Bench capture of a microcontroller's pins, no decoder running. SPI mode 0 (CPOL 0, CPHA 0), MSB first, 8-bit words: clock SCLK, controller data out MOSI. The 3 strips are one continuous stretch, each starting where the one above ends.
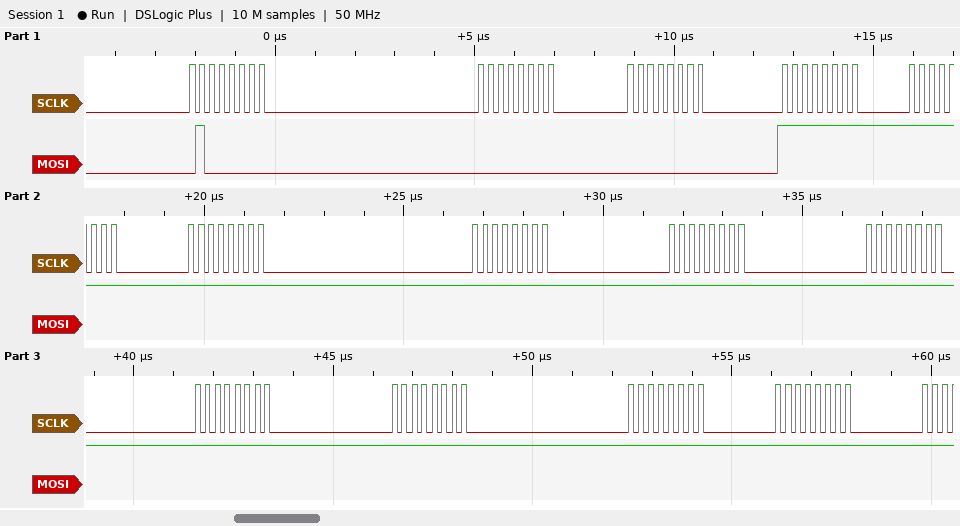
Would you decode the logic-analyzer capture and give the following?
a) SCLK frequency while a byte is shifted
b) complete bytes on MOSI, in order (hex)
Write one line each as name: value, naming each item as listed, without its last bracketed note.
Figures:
SCLK frequency while a byte is shifted: 4 MHz
complete bytes on MOSI, in order: 40 00 00 FF FF FF FF FF FF FF FF FF FF
